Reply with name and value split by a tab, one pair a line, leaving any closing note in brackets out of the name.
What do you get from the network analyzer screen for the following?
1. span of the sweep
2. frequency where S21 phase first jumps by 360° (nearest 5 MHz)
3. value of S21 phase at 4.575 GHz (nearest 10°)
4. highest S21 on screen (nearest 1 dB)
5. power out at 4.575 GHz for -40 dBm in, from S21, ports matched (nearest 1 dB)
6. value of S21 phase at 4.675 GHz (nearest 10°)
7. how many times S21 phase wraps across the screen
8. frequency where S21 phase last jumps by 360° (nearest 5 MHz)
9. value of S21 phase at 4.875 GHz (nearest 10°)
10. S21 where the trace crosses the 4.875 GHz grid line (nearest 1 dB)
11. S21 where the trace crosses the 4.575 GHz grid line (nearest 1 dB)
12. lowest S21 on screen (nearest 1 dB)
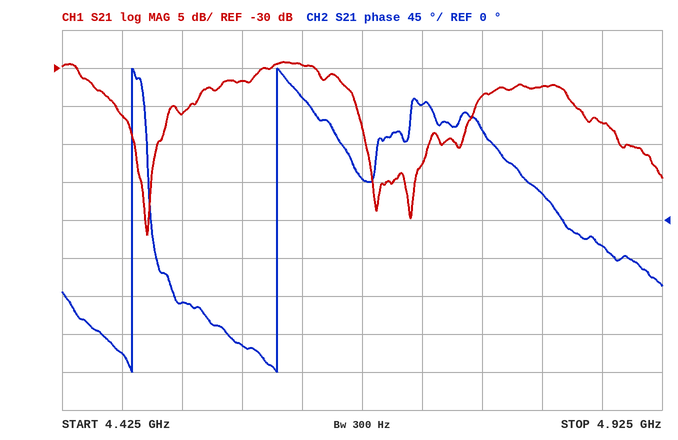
span of the sweep	500 MHz
frequency where S21 phase first jumps by 360°	4.485 GHz
value of S21 phase at 4.575 GHz	-150°
highest S21 on screen	-29 dB
power out at 4.575 GHz for -40 dBm in, from S21, ports matched	-72 dBm
value of S21 phase at 4.675 GHz	50°
how many times S21 phase wraps across the screen	2
frequency where S21 phase last jumps by 360°	4.605 GHz
value of S21 phase at 4.875 GHz	-30°
S21 where the trace crosses the 4.875 GHz grid line	-37 dB
S21 where the trace crosses the 4.575 GHz grid line	-32 dB
lowest S21 on screen	-52 dB
